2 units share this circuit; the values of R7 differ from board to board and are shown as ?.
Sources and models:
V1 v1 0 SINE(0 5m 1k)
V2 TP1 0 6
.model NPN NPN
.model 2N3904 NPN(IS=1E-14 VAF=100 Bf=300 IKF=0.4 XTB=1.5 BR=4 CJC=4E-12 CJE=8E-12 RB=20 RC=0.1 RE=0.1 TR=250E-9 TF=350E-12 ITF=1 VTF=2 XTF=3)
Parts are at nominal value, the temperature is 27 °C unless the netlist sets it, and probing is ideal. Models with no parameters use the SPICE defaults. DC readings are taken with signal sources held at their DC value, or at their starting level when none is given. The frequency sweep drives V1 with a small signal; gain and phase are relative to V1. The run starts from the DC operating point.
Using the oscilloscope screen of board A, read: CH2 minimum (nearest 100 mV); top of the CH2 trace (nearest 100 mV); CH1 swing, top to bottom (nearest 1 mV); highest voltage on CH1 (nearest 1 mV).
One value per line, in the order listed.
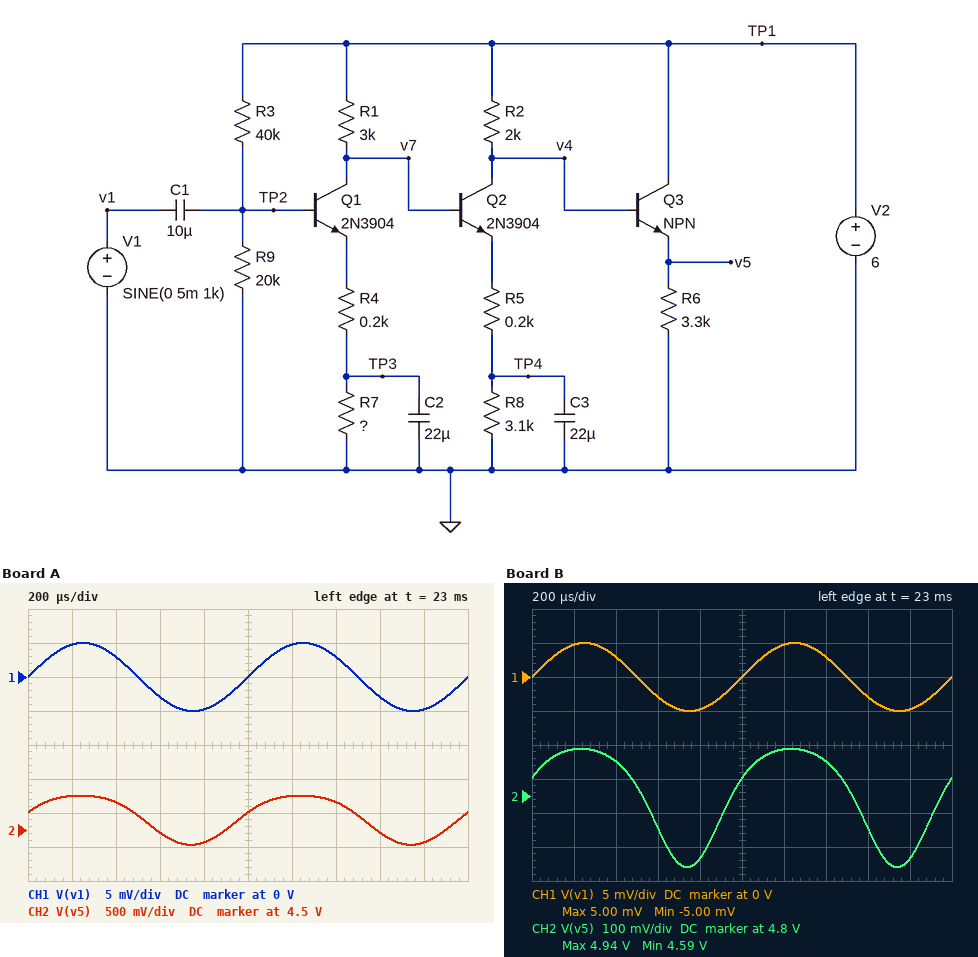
4.3 V
5.0 V
10 mV
5 mV
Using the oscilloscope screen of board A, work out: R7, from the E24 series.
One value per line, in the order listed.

620 Ω
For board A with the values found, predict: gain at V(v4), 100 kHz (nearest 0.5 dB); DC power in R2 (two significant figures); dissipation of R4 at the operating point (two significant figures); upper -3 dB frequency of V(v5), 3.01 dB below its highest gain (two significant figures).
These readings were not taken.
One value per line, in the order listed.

37.5 dB
130 µW
470 µW
1.1 MHz
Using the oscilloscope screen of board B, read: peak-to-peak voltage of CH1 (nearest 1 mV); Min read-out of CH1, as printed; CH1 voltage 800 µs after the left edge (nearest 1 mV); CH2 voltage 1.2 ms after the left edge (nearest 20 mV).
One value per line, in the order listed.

10 mV
-5.00 mV
-5 mV
4.94 V
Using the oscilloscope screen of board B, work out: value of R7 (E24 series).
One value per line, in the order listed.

510 Ω
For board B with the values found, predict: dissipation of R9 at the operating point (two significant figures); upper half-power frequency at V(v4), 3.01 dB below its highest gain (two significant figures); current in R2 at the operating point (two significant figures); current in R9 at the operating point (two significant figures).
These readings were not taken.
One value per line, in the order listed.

160 µW
330 kHz
200 µA
90 µA
